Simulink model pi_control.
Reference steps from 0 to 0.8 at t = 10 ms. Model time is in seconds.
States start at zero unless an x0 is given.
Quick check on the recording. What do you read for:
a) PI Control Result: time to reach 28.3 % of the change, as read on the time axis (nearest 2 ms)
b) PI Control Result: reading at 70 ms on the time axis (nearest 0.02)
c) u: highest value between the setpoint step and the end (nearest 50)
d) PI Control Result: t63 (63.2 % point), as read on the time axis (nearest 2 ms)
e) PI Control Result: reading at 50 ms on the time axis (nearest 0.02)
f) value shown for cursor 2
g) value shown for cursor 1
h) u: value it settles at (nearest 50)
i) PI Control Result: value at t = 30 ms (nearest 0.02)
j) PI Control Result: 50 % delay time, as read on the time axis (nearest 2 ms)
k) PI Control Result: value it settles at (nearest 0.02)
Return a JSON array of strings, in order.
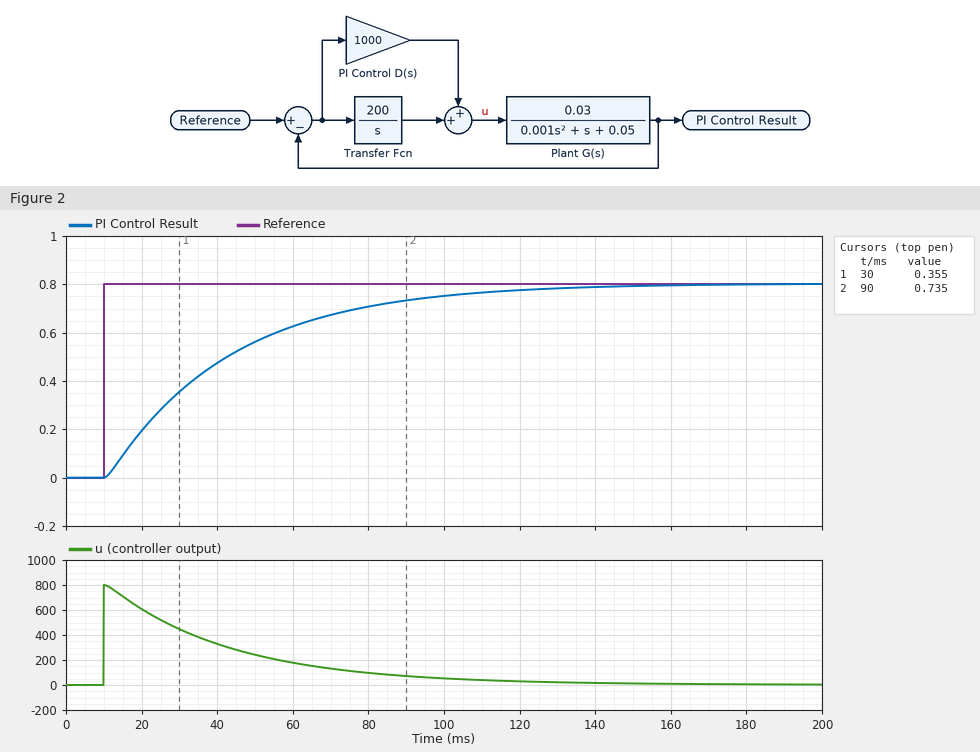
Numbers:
["22 ms", "0.68", "800", "44 ms", "0.56", "0.735", "0.355", "0", "0.36", "34 ms", "0.80"]
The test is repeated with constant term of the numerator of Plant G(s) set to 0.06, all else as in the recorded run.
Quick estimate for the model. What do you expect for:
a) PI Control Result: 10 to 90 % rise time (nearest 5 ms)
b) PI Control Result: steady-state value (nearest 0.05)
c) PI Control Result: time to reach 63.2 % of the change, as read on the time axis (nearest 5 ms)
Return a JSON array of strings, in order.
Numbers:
["35 ms", "0.80", "25 ms"]
